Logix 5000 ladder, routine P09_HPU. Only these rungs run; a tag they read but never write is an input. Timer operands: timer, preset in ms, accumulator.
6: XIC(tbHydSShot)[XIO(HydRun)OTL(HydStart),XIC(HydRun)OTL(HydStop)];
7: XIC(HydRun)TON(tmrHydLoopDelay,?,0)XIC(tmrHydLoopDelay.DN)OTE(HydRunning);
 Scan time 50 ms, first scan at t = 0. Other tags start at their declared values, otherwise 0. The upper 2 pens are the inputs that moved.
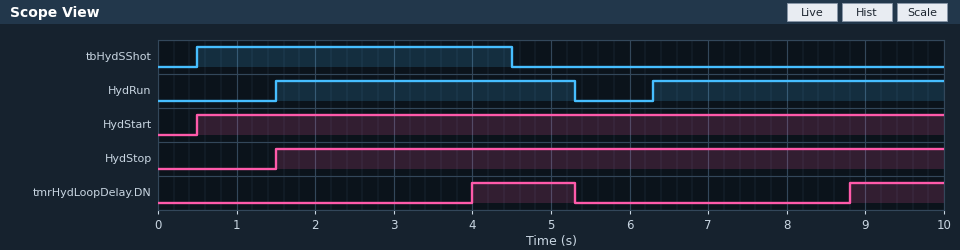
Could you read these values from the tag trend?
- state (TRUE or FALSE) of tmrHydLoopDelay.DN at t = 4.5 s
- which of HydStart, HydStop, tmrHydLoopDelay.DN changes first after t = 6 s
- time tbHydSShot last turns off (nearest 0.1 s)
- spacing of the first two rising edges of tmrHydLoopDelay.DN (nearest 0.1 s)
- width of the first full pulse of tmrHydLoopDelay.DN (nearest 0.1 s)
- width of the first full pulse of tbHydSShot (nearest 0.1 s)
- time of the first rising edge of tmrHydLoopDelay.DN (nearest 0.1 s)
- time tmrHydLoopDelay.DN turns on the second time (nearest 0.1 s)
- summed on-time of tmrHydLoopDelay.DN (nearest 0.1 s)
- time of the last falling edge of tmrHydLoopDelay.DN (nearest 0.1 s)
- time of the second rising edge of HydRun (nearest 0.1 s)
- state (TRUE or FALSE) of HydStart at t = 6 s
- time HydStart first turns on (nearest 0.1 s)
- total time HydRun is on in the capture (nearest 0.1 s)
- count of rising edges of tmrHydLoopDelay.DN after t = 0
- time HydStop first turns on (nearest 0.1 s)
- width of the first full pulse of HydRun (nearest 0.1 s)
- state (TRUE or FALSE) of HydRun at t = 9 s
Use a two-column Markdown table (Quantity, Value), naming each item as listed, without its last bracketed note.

| Quantity | Value |
|---|---|
| state (TRUE or FALSE) of tmrHydLoopDelay.DN at t = 4.5 s | TRUE |
| which of HydStart, HydStop, tmrHydLoopDelay.DN changes first after t = 6 s | tmrHydLoopDelay.DN |
| time tbHydSShot last turns off | 4.5 s |
| spacing of the first two rising edges of tmrHydLoopDelay.DN | 4.8 s |
| width of the first full pulse of tmrHydLoopDelay.DN | 1.3 s |
| width of the first full pulse of tbHydSShot | 4.0 s |
| time of the first rising edge of tmrHydLoopDelay.DN | 4.0 s |
| time tmrHydLoopDelay.DN turns on the second time | 8.8 s |
| summed on-time of tmrHydLoopDelay.DN | 2.5 s |
| time of the last falling edge of tmrHydLoopDelay.DN | 5.3 s |
| time of the second rising edge of HydRun | 6.3 s |
| state (TRUE or FALSE) of HydStart at t = 6 s | TRUE |
| time HydStart first turns on | 0.5 s |
| total time HydRun is on in the capture | 7.5 s |
| count of rising edges of tmrHydLoopDelay.DN after t = 0 | 2 |
| time HydStop first turns on | 1.5 s |
| width of the first full pulse of HydRun | 3.8 s |
| state (TRUE or FALSE) of HydRun at t = 9 s | TRUE |
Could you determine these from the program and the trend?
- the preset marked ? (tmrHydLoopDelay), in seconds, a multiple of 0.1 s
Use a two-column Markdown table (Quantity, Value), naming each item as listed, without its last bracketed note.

| Quantity | Value |
|---|---|
| the preset marked ? (tmrHydLoopDelay), in seconds, a multiple of 0.1 s | 2.5 s |
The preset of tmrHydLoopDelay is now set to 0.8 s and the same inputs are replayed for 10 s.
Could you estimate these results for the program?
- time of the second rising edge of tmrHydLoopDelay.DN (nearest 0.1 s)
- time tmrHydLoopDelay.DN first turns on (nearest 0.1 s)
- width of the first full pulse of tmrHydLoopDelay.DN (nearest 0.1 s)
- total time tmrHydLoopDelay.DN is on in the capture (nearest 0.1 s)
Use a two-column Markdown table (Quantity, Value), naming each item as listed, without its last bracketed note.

| Quantity | Value |
|---|---|
| time of the second rising edge of tmrHydLoopDelay.DN | 7.1 s |
| time tmrHydLoopDelay.DN first turns on | 2.3 s |
| width of the first full pulse of tmrHydLoopDelay.DN | 3.0 s |
| total time tmrHydLoopDelay.DN is on in the capture | 5.9 s |
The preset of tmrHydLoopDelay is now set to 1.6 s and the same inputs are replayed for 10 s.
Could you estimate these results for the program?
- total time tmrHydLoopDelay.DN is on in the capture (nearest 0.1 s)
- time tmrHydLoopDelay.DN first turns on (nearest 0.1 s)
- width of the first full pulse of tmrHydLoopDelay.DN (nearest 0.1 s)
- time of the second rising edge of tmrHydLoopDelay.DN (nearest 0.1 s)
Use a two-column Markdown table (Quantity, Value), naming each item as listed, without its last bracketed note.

| Quantity | Value |
|---|---|
| total time tmrHydLoopDelay.DN is on in the capture | 4.3 s |
| time tmrHydLoopDelay.DN first turns on | 3.1 s |
| width of the first full pulse of tmrHydLoopDelay.DN | 2.2 s |
| time of the second rising edge of tmrHydLoopDelay.DN | 7.9 s |
